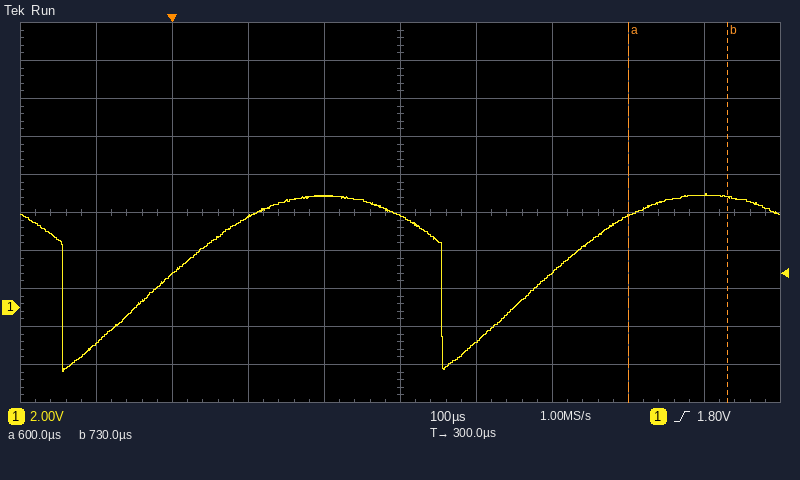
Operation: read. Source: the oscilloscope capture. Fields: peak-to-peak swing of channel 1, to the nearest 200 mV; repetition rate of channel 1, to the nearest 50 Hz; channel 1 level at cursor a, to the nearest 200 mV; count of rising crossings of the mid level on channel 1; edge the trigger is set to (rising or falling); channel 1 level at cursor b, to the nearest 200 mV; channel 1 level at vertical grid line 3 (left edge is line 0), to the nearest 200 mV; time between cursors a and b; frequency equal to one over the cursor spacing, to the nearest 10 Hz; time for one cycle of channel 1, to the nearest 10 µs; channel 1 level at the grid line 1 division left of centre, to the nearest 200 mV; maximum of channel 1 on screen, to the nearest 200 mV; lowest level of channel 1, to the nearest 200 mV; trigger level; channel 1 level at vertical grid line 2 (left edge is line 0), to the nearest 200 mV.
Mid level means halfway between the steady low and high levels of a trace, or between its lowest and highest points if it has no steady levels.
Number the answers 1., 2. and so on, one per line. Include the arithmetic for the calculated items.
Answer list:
1. 6.0 V − (-3.4 V) = 9.4 V
2. 1 / 500 µs ≈ 2.00 kHz
3. 4.8 V
4. 2
5. rising
6. 5.8 V
7. 4.8 V
8. 730 µs − (600 µs) = 130 µs
9. 1 / 130 µs ≈ 7.69 kHz
10. 500 µs
11. 5.8 V
12. 6.0 V
13. -3.4 V
14. 1.80 V
15. 1.8 V
